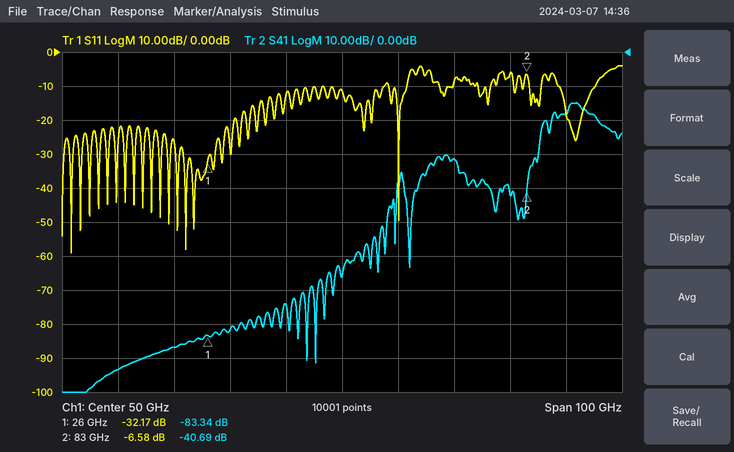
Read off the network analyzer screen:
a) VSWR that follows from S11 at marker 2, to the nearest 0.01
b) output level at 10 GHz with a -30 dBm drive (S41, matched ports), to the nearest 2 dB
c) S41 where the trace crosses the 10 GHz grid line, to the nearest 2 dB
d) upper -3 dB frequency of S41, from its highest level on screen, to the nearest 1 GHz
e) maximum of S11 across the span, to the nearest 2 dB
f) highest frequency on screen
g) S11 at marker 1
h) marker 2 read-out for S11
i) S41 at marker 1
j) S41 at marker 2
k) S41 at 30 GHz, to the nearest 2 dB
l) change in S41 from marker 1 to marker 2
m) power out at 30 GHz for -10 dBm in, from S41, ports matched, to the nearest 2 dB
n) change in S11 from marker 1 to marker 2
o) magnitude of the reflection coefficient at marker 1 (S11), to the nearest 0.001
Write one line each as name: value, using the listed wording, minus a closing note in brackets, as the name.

VSWR that follows from S11 at marker 2, to the nearest 0.01: 2.77
output level at 10 GHz with a -30 dBm drive (S41, matched ports), to the nearest 2 dB: -124 dBm
S41 where the trace crosses the 10 GHz grid line, to the nearest 2 dB: -94 dB
upper -3 dB frequency of S41, from its highest level on screen, to the nearest 1 GHz: 94 GHz
maximum of S11 across the span, to the nearest 2 dB: -4 dB
highest frequency on screen: 100 GHz
S11 at marker 1: -32.17 dB
marker 2 read-out for S11: -6.58 dB
S41 at marker 1: -83.34 dB
S41 at marker 2: -40.69 dB
S41 at 30 GHz, to the nearest 2 dB: -82 dB
change in S41 from marker 1 to marker 2: 42.65 dB
power out at 30 GHz for -10 dBm in, from S41, ports matched, to the nearest 2 dB: -92 dBm
change in S11 from marker 1 to marker 2: 25.59 dB
magnitude of the reflection coefficient at marker 1 (S11), to the nearest 0.001: 0.025
